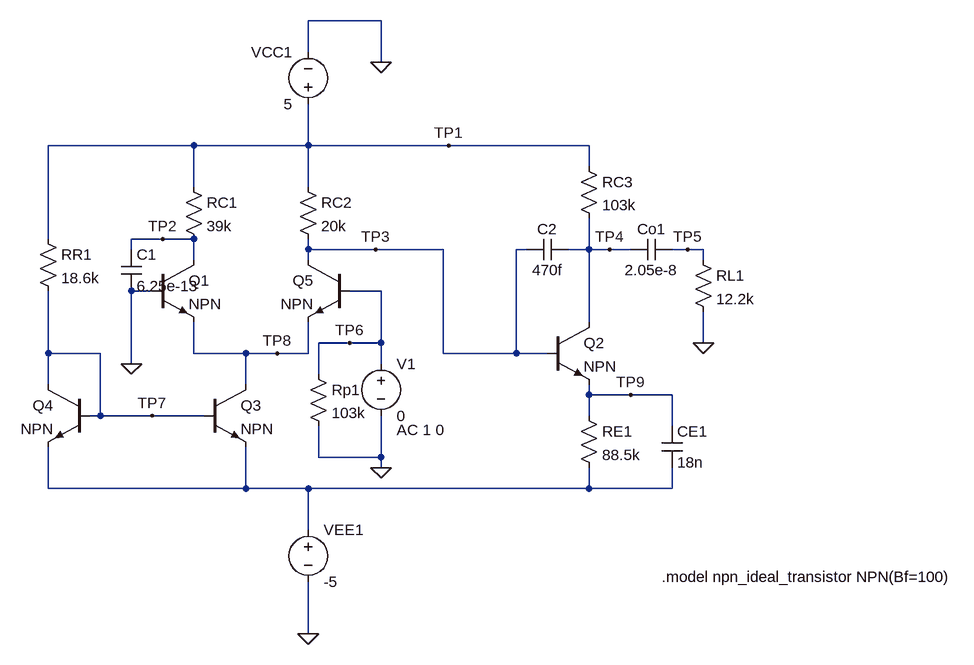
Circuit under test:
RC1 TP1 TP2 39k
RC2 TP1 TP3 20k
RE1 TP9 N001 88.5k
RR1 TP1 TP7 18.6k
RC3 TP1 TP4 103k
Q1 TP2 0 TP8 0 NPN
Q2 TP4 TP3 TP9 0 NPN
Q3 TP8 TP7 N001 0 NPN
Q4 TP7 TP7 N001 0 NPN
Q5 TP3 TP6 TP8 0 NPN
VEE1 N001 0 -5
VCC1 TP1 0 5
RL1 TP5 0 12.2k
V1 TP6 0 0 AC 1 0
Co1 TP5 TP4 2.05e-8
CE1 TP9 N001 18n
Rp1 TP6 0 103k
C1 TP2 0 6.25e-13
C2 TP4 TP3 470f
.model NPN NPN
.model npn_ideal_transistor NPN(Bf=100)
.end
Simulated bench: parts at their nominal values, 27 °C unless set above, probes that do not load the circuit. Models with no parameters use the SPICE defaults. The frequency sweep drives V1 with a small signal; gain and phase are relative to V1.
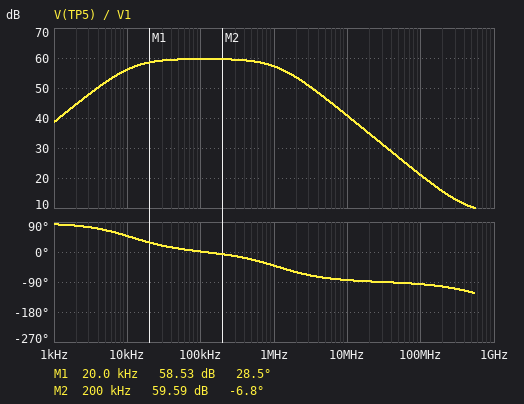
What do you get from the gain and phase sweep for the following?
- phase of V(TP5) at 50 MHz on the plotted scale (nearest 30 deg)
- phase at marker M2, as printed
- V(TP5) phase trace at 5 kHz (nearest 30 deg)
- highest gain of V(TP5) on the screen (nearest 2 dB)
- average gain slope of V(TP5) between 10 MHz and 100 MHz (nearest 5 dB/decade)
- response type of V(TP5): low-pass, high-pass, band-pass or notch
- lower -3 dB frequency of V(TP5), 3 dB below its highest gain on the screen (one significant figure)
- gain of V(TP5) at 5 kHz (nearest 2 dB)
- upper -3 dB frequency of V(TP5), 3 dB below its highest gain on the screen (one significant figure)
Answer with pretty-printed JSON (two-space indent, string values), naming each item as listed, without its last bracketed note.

{
  "phase of V(TP5) at 50 MHz on the plotted scale": "-90 deg",
  "phase at marker M2, as printed": "-6.8 deg",
  "V(TP5) phase trace at 5 kHz": "60 deg",
  "highest gain of V(TP5) on the screen": "60 dB",
  "average gain slope of V(TP5) between 10 MHz and 100 MHz": "-20 dB/decade",
  "response type of V(TP5): low-pass, high-pass, band-pass or notch": "band-pass",
  "lower -3 dB frequency of V(TP5), 3 dB below its highest gain on the screen": "10 kHz",
  "gain of V(TP5) at 5 kHz": "52 dB",
  "upper -3 dB frequency of V(TP5), 3 dB below its highest gain on the screen": "1 MHz"
}
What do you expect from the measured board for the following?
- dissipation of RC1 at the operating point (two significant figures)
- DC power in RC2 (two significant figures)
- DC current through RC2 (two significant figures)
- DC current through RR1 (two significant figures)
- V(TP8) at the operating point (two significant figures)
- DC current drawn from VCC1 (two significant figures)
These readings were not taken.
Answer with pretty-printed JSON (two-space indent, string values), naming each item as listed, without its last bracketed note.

{
  "dissipation of RC1 at the operating point": "830 µW",
  "DC power in RC2": "1.5 mW",
  "DC current through RC2": "270 µA",
  "DC current through RR1": "500 µA",
  "V(TP8) at the operating point": "-740 mV",
  "DC current drawn from VCC1": "960 µA"
}
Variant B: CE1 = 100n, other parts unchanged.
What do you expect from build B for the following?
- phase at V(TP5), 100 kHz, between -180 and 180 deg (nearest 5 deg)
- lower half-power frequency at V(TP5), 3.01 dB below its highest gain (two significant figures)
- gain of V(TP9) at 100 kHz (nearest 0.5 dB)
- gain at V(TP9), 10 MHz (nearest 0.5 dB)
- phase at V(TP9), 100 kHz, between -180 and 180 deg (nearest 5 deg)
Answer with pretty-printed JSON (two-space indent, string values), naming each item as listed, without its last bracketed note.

{
  "phase at V(TP5), 100 kHz, between -180 and 180 deg": "-5 deg",
  "lower half-power frequency at V(TP5), 3.01 dB below its highest gain": "2.0 kHz",
  "gain of V(TP9) at 100 kHz": "3.0 dB",
  "gain at V(TP9), 10 MHz": "-55.5 dB",
  "phase at V(TP9), 100 kHz, between -180 and 180 deg": "85 deg"
}
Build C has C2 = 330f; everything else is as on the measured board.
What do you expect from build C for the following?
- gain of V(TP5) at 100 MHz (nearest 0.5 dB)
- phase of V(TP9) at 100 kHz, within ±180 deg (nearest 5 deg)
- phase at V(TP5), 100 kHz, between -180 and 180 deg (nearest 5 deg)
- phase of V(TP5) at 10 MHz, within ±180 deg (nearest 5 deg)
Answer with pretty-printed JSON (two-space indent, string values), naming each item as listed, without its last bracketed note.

{
  "gain of V(TP5) at 100 MHz": "24.0 dB",
  "phase of V(TP9) at 100 kHz, within ±180 deg": "95 deg",
  "phase at V(TP5), 100 kHz, between -180 and 180 deg": "5 deg",
  "phase of V(TP5) at 10 MHz, within ±180 deg": "-80 deg"
}
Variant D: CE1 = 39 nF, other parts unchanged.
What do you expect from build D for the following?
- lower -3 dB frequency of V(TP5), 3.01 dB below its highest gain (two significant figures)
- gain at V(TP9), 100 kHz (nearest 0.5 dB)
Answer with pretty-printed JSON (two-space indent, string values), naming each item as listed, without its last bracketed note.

{
  "lower -3 dB frequency of V(TP5), 3.01 dB below its highest gain": "5.2 kHz",
  "gain at V(TP9), 100 kHz": "11.0 dB"
}
